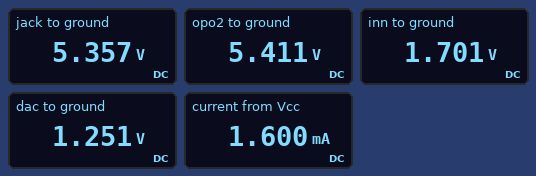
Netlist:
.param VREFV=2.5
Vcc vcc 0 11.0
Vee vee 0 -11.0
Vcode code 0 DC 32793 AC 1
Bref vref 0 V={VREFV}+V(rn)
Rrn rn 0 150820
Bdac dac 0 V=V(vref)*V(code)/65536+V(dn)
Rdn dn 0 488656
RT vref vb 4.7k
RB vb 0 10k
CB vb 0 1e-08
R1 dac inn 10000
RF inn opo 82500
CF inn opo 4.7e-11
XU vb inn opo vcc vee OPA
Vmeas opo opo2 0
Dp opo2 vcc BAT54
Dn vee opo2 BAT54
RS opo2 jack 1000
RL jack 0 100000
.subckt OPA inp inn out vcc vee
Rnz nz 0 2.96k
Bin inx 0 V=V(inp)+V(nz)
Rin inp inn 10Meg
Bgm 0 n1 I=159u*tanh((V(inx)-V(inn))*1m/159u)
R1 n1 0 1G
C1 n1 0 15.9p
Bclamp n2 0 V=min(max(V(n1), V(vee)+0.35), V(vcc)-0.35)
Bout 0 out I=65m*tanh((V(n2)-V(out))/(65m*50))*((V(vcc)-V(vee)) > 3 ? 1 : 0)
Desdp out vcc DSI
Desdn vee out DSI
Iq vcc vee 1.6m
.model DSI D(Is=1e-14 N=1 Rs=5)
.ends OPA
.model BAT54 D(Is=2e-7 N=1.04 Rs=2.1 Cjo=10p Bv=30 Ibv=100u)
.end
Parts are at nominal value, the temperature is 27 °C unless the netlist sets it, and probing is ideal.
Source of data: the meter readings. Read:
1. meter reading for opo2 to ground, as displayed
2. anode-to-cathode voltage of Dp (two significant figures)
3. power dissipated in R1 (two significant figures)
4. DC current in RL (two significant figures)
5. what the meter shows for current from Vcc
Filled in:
5.411 V
-5.6 V
20 µW
54 µA
1.600 mA
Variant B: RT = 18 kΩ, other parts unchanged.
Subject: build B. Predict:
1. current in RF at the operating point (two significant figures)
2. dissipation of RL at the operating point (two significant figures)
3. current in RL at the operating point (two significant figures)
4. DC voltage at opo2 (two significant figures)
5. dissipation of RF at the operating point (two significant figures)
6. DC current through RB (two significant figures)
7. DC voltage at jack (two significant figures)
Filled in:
36 µA
42 µW
20 µA
-2.1 V
110 µW
89 µA
-2.0 V
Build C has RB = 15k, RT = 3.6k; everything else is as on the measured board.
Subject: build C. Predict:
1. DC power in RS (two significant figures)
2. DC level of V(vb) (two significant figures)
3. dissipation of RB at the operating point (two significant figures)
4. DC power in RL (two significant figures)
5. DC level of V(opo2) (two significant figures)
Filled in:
6.8 µW
2.0 V
270 µW
680 µW
8.3 V
